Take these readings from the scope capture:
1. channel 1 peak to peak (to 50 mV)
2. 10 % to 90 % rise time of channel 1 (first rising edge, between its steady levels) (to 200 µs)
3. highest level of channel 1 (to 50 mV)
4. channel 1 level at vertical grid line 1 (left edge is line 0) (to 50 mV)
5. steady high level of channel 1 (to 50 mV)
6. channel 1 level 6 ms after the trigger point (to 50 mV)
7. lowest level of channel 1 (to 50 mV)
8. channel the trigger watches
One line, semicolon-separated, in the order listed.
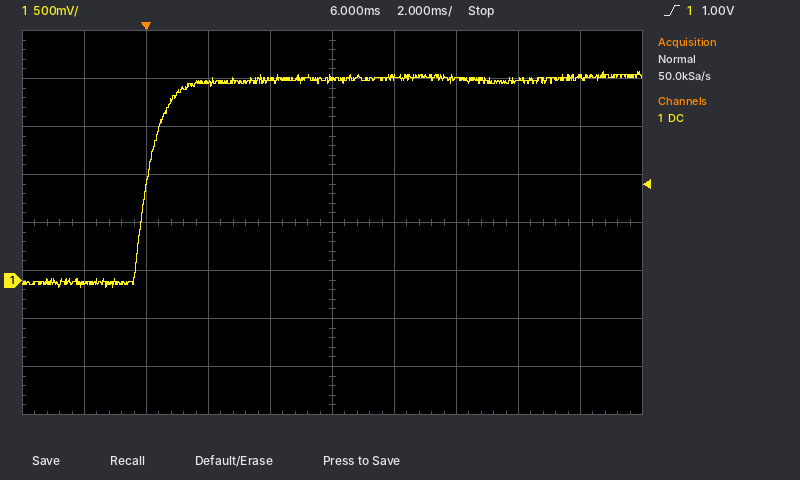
2.25 V; 1.2 ms; 2.15 V; -50 mV; 2.10 V; 2.10 V; -100 mV; channel 1
